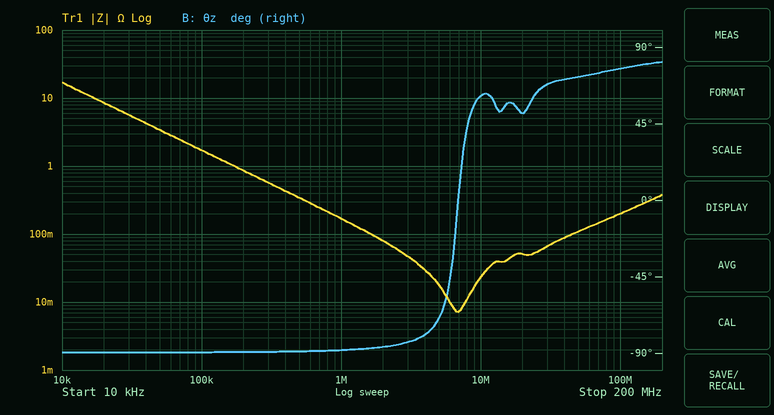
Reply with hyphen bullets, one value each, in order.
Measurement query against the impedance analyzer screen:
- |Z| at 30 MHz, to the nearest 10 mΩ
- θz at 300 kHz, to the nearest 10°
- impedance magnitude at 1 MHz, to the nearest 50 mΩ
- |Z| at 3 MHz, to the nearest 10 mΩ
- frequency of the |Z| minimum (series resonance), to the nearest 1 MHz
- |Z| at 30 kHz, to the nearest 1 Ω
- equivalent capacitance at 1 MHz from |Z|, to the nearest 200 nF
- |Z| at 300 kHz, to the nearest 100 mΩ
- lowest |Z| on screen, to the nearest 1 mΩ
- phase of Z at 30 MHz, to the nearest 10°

- 70 mΩ
- -90°
- 150 mΩ
- 50 mΩ
- 7 MHz
- 6 Ω
- 1.0 µF
- 600 mΩ
- 7 mΩ
- 70°
